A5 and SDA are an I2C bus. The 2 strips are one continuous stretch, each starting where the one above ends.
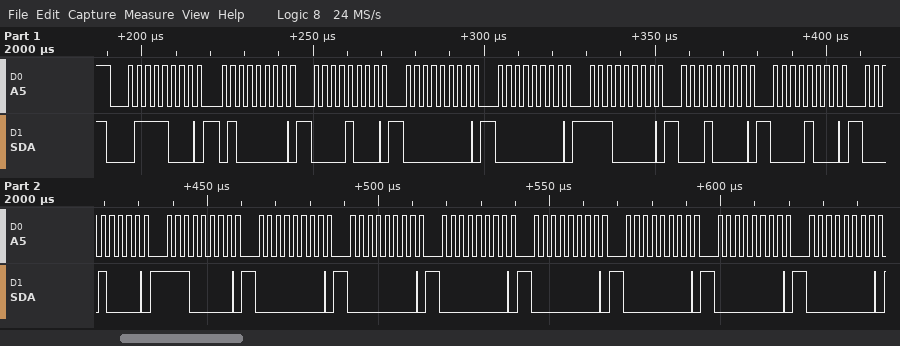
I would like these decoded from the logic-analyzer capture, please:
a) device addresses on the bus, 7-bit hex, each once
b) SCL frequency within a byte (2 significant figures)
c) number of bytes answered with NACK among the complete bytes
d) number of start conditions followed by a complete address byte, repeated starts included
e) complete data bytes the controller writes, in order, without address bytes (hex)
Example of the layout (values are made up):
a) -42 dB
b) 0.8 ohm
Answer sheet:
a) 0x3C
b) 400 kHz
c) 0
d) 1
e) 40 08 00 00 E0 10 08 10 E0 00 00 00 00 00 00 00
